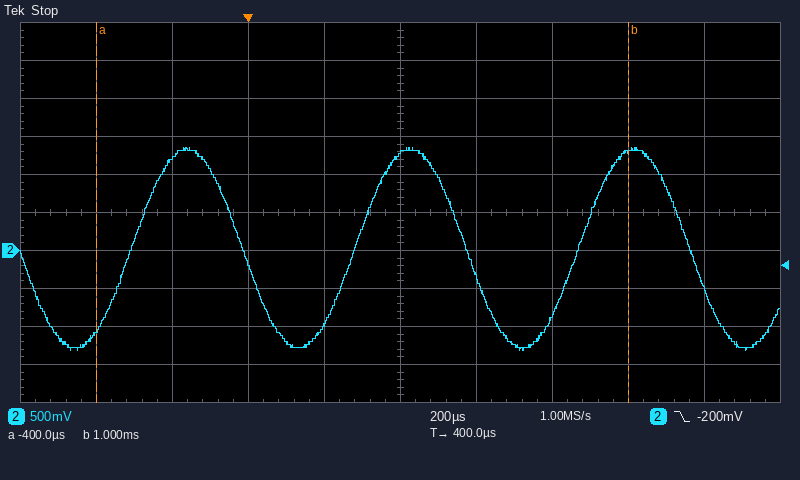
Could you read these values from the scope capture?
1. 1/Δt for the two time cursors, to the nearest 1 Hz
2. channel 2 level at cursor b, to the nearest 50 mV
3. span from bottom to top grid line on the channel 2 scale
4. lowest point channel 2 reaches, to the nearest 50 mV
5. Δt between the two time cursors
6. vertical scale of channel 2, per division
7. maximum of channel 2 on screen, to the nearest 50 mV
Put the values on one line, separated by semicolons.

714 Hz; 1.30 V; 5 V; -1.30 V; 1.40 ms; 500 mV; 1.35 V
